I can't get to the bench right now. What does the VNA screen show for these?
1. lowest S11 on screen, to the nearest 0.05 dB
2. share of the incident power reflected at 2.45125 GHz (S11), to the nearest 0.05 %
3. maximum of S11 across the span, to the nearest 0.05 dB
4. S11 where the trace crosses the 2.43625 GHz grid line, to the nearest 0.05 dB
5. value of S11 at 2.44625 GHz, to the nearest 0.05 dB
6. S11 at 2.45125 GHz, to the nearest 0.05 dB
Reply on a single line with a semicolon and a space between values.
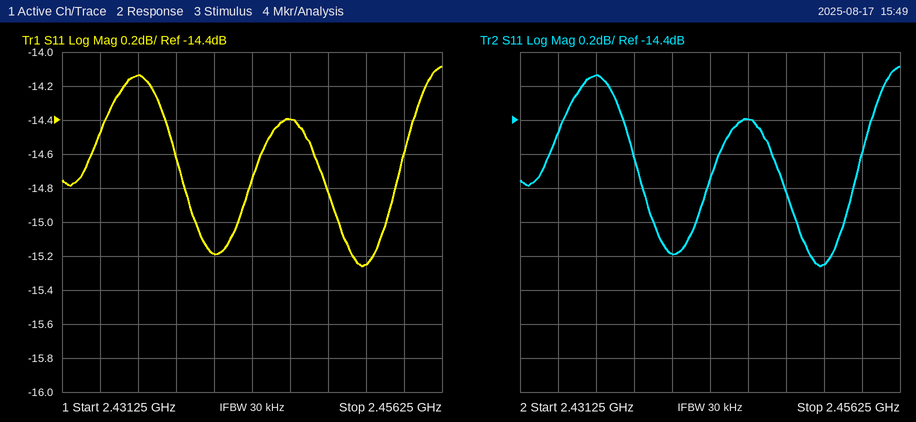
-15.25 dB; 3.00 %; -14.10 dB; -14.15 dB; -14.40 dB; -15.25 dB
